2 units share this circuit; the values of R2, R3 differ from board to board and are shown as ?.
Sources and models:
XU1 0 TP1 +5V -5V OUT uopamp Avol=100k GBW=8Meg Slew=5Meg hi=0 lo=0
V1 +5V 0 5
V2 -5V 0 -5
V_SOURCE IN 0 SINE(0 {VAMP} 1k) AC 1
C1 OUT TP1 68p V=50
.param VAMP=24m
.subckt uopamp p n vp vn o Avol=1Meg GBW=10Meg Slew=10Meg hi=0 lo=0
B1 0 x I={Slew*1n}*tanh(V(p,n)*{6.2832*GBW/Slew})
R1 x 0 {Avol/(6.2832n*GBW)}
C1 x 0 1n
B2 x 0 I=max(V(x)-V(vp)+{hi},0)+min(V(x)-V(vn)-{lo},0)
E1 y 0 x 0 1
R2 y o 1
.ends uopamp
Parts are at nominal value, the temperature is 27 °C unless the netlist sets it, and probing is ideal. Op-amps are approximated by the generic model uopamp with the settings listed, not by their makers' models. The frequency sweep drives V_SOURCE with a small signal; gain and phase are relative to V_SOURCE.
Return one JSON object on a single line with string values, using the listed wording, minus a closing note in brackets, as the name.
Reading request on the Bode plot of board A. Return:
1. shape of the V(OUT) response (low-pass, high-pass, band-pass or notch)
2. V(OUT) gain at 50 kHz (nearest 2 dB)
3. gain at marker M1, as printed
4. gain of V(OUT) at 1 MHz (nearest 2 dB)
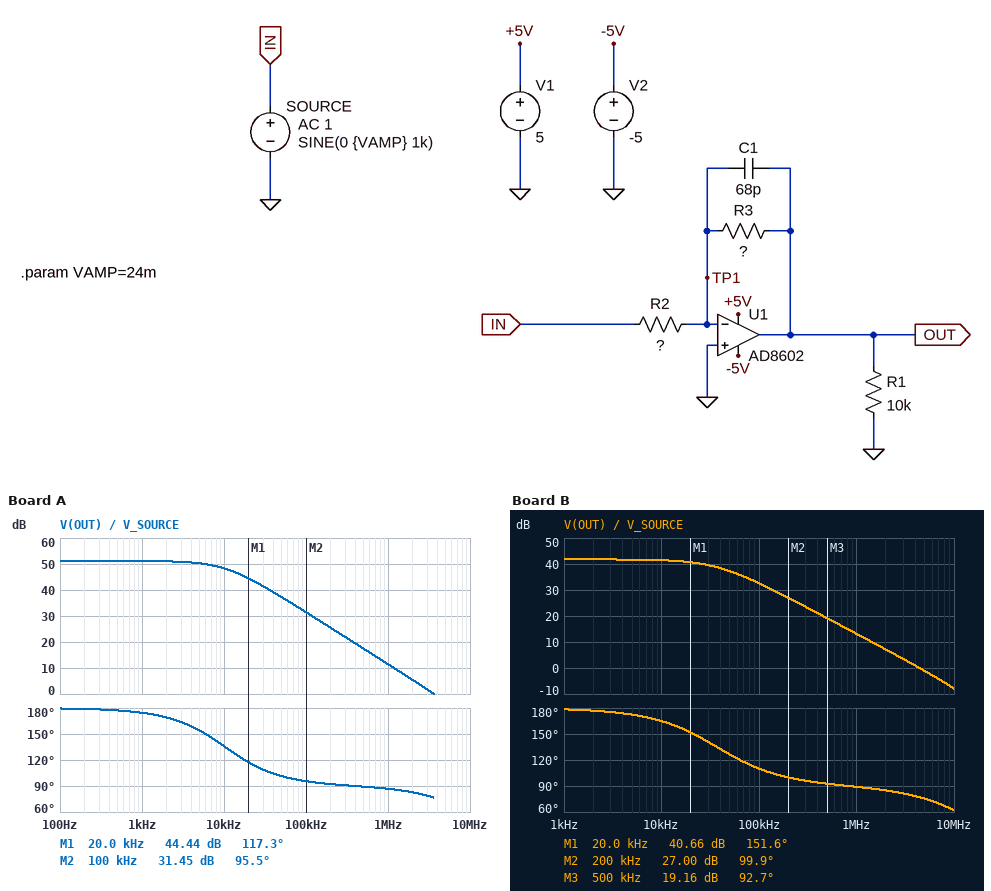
{"shape of the V(OUT) response": "low-pass", "V(OUT) gain at 50 kHz": "38 dB", "gain at marker M1, as printed": "44.44 dB", "gain of V(OUT) at 1 MHz": "12 dB"}
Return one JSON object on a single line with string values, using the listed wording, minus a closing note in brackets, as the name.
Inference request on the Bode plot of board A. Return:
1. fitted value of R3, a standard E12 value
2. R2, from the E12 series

{"fitted value of R3, a standard E12 value": "120 kΩ", "R2, from the E12 series": "330 Ω"}
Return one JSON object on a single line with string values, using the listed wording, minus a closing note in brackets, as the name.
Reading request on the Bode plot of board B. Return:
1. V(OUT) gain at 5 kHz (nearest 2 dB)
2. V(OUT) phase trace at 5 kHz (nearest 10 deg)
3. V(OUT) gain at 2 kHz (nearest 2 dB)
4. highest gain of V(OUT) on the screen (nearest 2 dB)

{"V(OUT) gain at 5 kHz": "42 dB", "V(OUT) phase trace at 5 kHz": "170 deg", "V(OUT) gain at 2 kHz": "42 dB", "highest gain of V(OUT) on the screen": "42 dB"}
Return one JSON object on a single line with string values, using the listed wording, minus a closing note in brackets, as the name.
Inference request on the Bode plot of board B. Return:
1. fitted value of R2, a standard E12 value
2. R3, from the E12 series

{"fitted value of R2, a standard E12 value": "220 Ω", "R3, from the E12 series": "27 kΩ"}
